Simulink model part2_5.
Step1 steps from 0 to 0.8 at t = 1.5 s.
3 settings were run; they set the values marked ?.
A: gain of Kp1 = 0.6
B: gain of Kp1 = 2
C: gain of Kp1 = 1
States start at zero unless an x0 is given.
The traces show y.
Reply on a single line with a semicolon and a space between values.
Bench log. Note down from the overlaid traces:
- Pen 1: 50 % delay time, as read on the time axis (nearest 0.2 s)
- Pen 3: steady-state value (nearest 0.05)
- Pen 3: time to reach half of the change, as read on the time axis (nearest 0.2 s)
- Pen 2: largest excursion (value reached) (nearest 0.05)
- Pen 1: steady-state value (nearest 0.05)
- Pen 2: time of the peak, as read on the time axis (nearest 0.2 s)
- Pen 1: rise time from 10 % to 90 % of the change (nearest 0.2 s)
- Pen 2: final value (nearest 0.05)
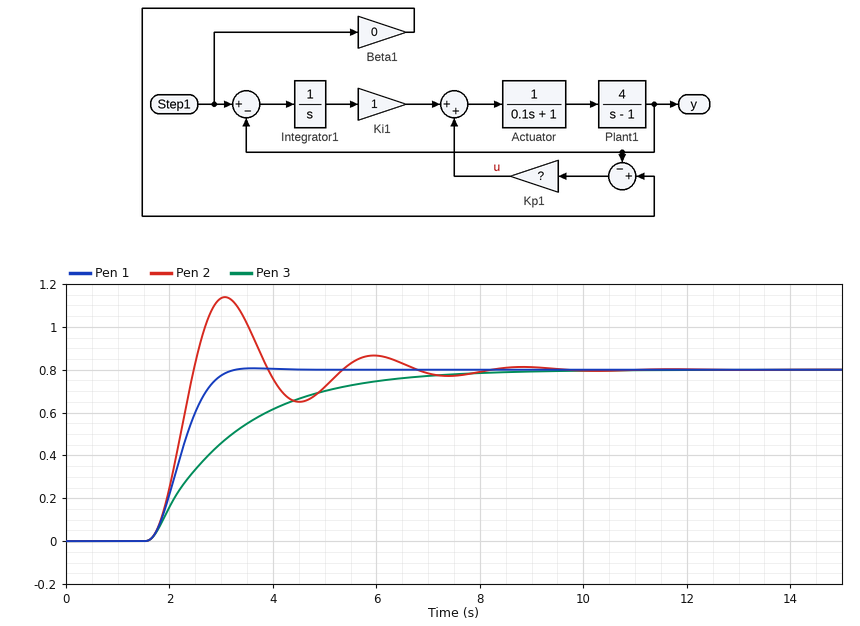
2.2 s; 0.80; 2.8 s; 1.15; 0.80; 3.0 s; 1.0 s; 0.80
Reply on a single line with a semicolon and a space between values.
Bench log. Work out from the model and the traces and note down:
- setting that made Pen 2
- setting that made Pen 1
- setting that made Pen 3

A; C; B
